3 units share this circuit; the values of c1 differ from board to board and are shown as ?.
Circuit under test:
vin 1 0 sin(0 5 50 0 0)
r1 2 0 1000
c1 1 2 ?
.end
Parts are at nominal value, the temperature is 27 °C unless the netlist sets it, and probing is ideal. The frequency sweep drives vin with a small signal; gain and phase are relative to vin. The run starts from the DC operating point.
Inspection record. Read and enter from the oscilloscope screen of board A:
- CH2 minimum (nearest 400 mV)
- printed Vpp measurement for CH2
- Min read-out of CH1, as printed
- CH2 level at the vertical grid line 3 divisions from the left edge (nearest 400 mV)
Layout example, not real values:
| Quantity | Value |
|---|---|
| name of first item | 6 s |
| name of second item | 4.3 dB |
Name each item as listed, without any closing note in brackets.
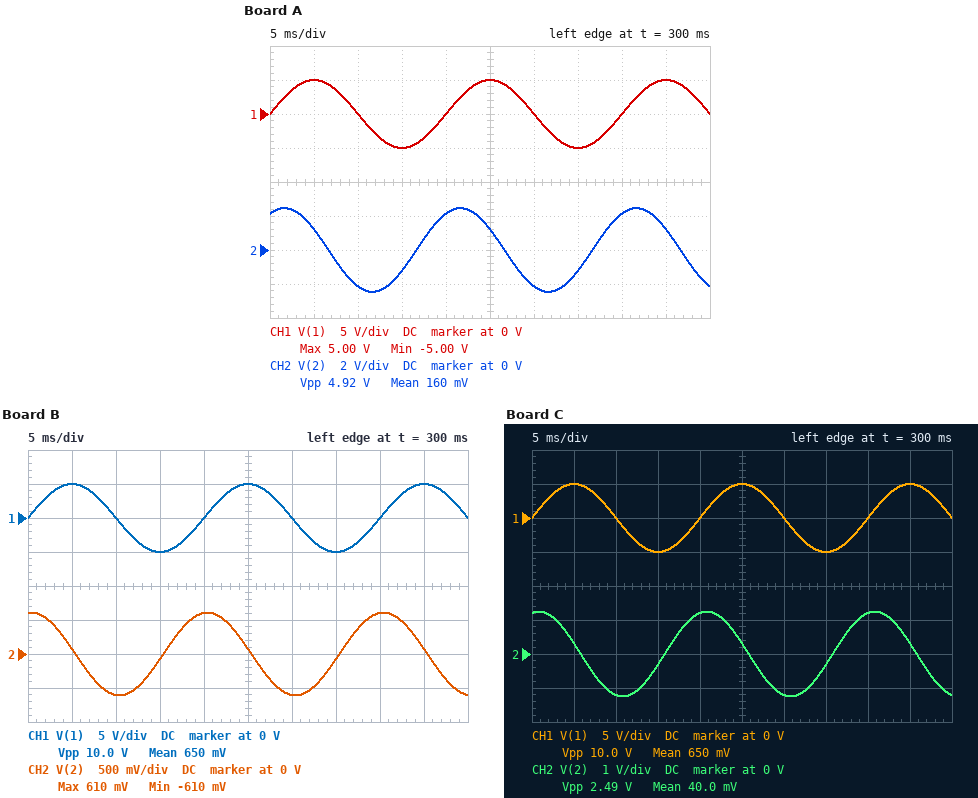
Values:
| Quantity | Value |
|---|---|
| CH2 minimum | -2.4 V |
| printed Vpp measurement for CH2 | 4.92 V |
| Min read-out of CH1, as printed | -5.00 V |
| CH2 level at the vertical grid line 3 divisions from the left edge | -1.2 V |
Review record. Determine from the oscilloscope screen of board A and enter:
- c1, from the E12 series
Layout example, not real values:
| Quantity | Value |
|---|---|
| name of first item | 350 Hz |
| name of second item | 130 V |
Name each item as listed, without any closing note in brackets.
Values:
| Quantity | Value |
|---|---|
| c1, from the E12 series | 1.8 µF |
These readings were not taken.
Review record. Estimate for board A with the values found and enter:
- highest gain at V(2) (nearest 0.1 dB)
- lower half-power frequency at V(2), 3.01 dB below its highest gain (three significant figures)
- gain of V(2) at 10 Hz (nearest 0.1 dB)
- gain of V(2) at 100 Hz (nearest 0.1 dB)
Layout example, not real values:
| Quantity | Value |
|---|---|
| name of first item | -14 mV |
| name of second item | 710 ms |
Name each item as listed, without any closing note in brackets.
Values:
| Quantity | Value |
|---|---|
| highest gain at V(2) | 0 dB |
| lower half-power frequency at V(2), 3.01 dB below its highest gain | 88.4 Hz |
| gain of V(2) at 10 Hz | -19.0 dB |
| gain of V(2) at 100 Hz | -2.5 dB |
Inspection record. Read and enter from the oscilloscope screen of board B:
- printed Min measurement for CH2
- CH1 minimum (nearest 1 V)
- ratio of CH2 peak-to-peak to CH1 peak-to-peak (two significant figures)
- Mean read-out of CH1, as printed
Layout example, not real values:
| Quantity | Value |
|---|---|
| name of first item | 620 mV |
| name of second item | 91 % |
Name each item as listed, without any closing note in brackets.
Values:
| Quantity | Value |
|---|---|
| printed Min measurement for CH2 | -610 mV |
| CH1 minimum | -5 V |
| ratio of CH2 peak-to-peak to CH1 peak-to-peak | 0.12 |
| Mean read-out of CH1, as printed | 650 mV |
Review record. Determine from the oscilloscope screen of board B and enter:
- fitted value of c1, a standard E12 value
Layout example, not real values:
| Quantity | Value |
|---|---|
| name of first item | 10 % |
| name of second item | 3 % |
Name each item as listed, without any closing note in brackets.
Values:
| Quantity | Value |
|---|---|
| fitted value of c1, a standard E12 value | 390 nF |
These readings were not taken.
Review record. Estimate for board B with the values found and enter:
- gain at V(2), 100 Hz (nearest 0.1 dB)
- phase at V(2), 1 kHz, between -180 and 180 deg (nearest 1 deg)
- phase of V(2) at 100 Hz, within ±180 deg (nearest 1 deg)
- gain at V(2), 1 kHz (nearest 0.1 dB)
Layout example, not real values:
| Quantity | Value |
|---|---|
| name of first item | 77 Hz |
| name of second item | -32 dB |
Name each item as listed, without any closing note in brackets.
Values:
| Quantity | Value |
|---|---|
| gain at V(2), 100 Hz | -12.5 dB |
| phase at V(2), 1 kHz, between -180 and 180 deg | 22 deg |
| phase of V(2) at 100 Hz, within ±180 deg | 76 deg |
| gain at V(2), 1 kHz | -0.7 dB |
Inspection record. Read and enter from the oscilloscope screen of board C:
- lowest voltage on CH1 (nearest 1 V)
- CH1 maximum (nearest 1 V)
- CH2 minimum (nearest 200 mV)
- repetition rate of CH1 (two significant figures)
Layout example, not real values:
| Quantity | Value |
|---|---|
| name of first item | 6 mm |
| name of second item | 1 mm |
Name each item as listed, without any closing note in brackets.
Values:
| Quantity | Value |
|---|---|
| lowest voltage on CH1 | -5 V |
| CH1 maximum | 5 V |
| CH2 minimum | -1.2 V |
| repetition rate of CH1 | 50 Hz |
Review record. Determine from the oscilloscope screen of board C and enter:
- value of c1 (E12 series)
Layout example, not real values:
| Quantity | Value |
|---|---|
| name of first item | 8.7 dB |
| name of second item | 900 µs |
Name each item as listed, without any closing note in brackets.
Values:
| Quantity | Value |
|---|---|
| value of c1 | 820 nF |
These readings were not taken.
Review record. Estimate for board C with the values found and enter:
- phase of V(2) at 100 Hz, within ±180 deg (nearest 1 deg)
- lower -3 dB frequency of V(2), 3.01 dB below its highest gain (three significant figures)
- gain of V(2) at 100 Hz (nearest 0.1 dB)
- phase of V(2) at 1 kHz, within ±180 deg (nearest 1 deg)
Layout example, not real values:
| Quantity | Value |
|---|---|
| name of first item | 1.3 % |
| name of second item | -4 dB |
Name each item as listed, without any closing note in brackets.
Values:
| Quantity | Value |
|---|---|
| phase of V(2) at 100 Hz, within ±180 deg | 63 deg |
| lower -3 dB frequency of V(2), 3.01 dB below its highest gain | 194 Hz |
| gain of V(2) at 100 Hz | -6.8 dB |
| phase of V(2) at 1 kHz, within ±180 deg | 11 deg |
